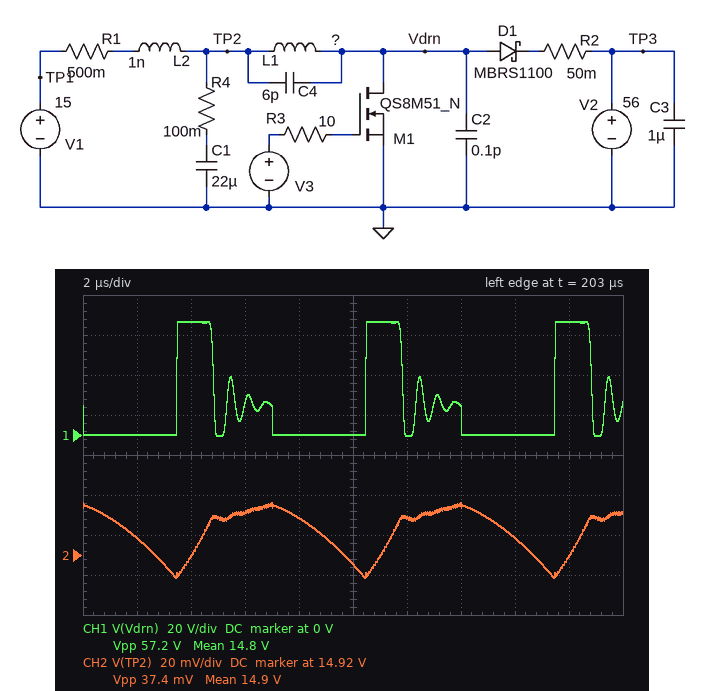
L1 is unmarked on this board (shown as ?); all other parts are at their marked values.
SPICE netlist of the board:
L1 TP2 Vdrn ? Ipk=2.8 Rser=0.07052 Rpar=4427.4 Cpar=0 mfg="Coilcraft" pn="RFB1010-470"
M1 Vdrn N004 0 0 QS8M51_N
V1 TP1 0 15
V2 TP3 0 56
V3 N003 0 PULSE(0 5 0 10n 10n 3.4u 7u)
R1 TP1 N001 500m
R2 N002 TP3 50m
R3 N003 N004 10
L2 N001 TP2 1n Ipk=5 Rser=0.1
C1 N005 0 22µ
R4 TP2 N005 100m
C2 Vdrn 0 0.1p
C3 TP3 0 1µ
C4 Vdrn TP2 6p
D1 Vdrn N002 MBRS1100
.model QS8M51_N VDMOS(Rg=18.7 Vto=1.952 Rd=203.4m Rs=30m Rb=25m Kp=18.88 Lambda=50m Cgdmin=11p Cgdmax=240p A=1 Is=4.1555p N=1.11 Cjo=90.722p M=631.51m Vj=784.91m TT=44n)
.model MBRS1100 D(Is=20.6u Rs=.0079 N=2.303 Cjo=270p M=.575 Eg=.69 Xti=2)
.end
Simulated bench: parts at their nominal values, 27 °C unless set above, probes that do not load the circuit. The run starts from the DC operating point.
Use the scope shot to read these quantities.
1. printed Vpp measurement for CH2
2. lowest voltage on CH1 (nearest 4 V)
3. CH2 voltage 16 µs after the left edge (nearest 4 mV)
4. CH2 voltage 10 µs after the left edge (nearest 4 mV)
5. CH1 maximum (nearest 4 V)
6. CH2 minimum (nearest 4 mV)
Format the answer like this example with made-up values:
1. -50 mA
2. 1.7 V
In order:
1. 37.4 mV
2. 0 V
3. 14.928 V
4. 14.916 V
5. 56 V
6. 14.908 V
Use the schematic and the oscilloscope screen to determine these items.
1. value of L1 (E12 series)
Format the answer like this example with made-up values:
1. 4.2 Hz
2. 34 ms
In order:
1. 150 µH
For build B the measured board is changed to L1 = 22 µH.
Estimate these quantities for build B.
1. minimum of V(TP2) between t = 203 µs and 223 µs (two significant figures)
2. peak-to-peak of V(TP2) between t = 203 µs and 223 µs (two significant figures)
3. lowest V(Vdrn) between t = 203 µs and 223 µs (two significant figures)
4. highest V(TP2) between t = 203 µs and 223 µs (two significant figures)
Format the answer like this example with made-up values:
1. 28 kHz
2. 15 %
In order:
1. 14 V
2. 240 mV
3. -660 mV
4. 15 V
